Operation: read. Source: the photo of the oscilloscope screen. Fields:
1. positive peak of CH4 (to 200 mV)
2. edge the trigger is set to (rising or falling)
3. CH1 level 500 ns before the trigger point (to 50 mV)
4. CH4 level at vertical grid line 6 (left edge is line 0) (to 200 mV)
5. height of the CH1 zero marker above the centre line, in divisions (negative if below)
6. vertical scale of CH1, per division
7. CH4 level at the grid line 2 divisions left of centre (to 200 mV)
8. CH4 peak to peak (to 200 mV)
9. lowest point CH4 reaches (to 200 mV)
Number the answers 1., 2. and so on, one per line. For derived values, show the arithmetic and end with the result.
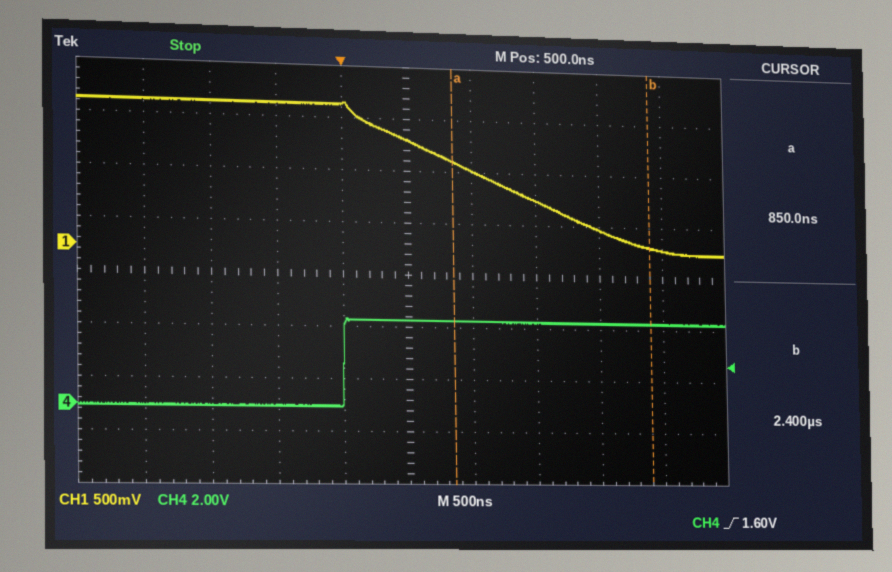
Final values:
1. 3.4 V
2. rising
3. 1.40 V
4. 3.2 V
5. +0.5 div
6. 500 mV
7. 0.0 V
8. 3.4 V − (0.0 V) = 3.4 V
9. 0.0 V
